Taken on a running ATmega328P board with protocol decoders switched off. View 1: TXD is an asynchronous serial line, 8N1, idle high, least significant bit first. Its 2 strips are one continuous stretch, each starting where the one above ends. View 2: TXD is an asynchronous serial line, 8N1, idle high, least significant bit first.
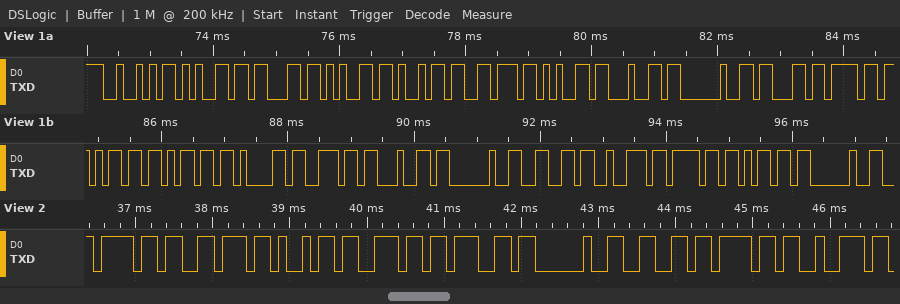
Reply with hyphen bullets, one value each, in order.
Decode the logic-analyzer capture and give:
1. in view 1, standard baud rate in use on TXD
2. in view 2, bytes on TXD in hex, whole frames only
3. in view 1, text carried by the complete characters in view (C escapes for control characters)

- 9600 baud
- 6F 76 69 6E 67 20 66 6F 72
- "Received command from "
